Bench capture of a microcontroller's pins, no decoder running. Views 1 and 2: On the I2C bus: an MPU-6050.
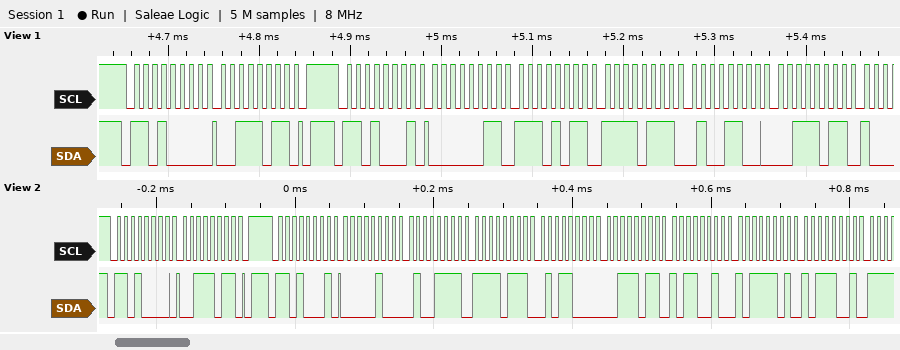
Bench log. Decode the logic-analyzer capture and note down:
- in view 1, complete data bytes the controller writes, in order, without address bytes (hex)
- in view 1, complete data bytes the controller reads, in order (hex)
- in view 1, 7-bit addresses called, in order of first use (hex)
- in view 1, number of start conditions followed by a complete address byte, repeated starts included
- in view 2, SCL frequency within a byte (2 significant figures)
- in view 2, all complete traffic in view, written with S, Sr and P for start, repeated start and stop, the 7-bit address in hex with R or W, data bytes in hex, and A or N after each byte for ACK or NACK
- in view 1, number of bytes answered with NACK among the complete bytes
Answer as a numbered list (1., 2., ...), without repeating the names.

1. 3B
2. 03 EB F7 4C 3B
3. 0x68
4. 2
5. 100 kHz
6. S 68W A 3B A P S 68R A 04 A 4F A F7 A 58 A 3B A B2 A BD A B9 A
7. 0
